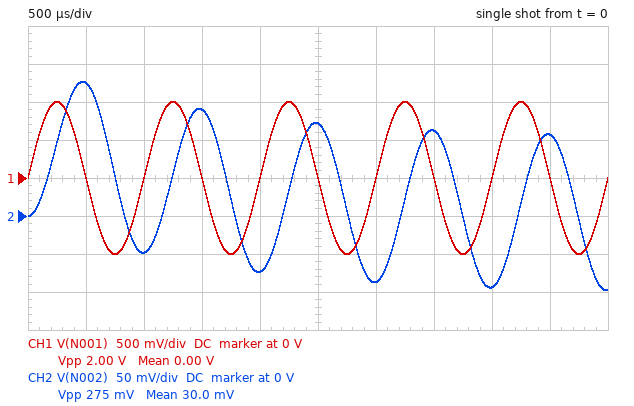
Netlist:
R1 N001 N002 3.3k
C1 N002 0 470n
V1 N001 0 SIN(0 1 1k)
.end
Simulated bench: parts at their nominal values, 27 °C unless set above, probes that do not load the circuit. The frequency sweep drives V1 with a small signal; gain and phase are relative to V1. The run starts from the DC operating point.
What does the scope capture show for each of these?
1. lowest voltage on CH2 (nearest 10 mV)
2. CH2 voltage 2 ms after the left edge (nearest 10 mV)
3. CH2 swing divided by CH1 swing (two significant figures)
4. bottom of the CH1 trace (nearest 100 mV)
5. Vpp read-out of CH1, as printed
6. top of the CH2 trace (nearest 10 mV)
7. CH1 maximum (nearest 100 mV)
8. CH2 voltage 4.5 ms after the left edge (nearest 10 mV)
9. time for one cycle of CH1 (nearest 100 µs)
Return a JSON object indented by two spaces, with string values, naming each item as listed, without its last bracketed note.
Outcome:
{
  "lowest voltage on CH2": "-100 mV",
  "CH2 voltage 2 ms after the left edge": "-70 mV",
  "CH2 swing divided by CH1 swing": "0.14",
  "bottom of the CH1 trace": "-1.0 V",
  "Vpp read-out of CH1, as printed": "2.00 V",
  "top of the CH2 trace": "180 mV",
  "CH1 maximum": "1.0 V",
  "CH2 voltage 4.5 ms after the left edge": "110 mV",
  "time for one cycle of CH1": "1.0 ms"
}
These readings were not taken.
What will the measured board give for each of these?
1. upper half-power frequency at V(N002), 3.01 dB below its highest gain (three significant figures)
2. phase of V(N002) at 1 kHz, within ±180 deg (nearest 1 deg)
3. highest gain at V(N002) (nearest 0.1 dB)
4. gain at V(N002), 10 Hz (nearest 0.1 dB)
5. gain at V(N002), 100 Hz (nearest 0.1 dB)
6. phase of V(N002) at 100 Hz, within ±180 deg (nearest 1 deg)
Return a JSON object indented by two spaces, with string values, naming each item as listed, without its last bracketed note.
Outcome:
{
  "upper half-power frequency at V(N002), 3.01 dB below its highest gain": "103 Hz",
  "phase of V(N002) at 1 kHz, within ±180 deg": "-84 deg",
  "highest gain at V(N002)": "0 dB",
  "gain at V(N002), 10 Hz": "0 dB",
  "gain at V(N002), 100 Hz": "-2.9 dB",
  "phase of V(N002) at 100 Hz, within ±180 deg": "-44 deg"
}
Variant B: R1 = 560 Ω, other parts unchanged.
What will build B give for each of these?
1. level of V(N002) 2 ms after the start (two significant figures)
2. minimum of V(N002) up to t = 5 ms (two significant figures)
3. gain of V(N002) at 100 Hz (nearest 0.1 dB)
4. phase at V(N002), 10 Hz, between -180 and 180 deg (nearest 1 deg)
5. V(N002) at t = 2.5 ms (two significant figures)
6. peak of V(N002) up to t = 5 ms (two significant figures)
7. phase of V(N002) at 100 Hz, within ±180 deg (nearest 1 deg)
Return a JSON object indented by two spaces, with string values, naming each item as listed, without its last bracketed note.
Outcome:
{
  "level of V(N002) 2 ms after the start": "-440 mV",
  "minimum of V(N002) up to t = 5 ms": "-520 mV",
  "gain of V(N002) at 100 Hz": "-0.1 dB",
  "phase at V(N002), 10 Hz, between -180 and 180 deg": "-1 deg",
  "V(N002) at t = 2.5 ms": "440 mV",
  "peak of V(N002) up to t = 5 ms": "610 mV",
  "phase of V(N002) at 100 Hz, within ±180 deg": "-9 deg"
}
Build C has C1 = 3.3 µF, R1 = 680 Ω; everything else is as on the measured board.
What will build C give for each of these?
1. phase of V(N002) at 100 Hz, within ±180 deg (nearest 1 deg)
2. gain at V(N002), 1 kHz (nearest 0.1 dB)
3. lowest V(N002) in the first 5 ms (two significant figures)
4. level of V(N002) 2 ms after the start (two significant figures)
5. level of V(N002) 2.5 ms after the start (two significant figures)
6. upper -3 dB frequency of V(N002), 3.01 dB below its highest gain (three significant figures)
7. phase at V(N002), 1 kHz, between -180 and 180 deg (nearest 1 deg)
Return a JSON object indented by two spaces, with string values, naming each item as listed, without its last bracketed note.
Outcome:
{
  "phase of V(N002) at 100 Hz, within ±180 deg": "-55 deg",
  "gain at V(N002), 1 kHz": "-23.0 dB",
  "lowest V(N002) in the first 5 ms": "-63 mV",
  "level of V(N002) 2 ms after the start": "-42 mV",
  "level of V(N002) 2.5 ms after the start": "94 mV",
  "upper -3 dB frequency of V(N002), 3.01 dB below its highest gain": "70.9 Hz",
  "phase at V(N002), 1 kHz, between -180 and 180 deg": "-86 deg"
}
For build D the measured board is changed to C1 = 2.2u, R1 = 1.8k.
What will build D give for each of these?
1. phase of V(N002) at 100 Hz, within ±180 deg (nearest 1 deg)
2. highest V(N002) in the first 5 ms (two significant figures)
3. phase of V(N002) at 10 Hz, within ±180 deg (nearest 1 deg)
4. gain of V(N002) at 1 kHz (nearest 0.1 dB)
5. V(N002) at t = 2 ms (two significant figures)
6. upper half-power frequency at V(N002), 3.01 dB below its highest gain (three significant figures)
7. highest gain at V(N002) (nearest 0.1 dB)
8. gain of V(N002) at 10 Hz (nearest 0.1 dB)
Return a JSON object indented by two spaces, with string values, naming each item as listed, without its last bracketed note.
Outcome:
{
  "phase of V(N002) at 100 Hz, within ±180 deg": "-68 deg",
  "highest V(N002) in the first 5 ms": "76 mV",
  "phase of V(N002) at 10 Hz, within ±180 deg": "-14 deg",
  "gain of V(N002) at 1 kHz": "-27.9 dB",
  "V(N002) at t = 2 ms": "-16 mV",
  "upper half-power frequency at V(N002), 3.01 dB below its highest gain": "40.2 Hz",
  "highest gain at V(N002)": "0 dB",
  "gain of V(N002) at 10 Hz": "-0.3 dB"
}
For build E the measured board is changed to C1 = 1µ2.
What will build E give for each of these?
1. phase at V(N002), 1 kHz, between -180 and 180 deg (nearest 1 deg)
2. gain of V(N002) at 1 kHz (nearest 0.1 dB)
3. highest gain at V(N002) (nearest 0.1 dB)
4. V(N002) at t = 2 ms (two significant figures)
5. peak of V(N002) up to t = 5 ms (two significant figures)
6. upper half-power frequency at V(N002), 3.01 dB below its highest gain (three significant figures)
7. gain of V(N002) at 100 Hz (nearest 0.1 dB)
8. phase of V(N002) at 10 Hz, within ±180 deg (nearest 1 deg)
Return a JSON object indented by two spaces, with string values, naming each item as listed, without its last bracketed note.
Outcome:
{
  "phase at V(N002), 1 kHz, between -180 and 180 deg": "-88 deg",
  "gain of V(N002) at 1 kHz": "-27.9 dB",
  "highest gain at V(N002)": "0 dB",
  "V(N002) at t = 2 ms": "-16 mV",
  "peak of V(N002) up to t = 5 ms": "76 mV",
  "upper half-power frequency at V(N002), 3.01 dB below its highest gain": "40.2 Hz",
  "gain of V(N002) at 100 Hz": "-8.6 dB",
  "phase of V(N002) at 10 Hz, within ±180 deg": "-14 deg"
}
